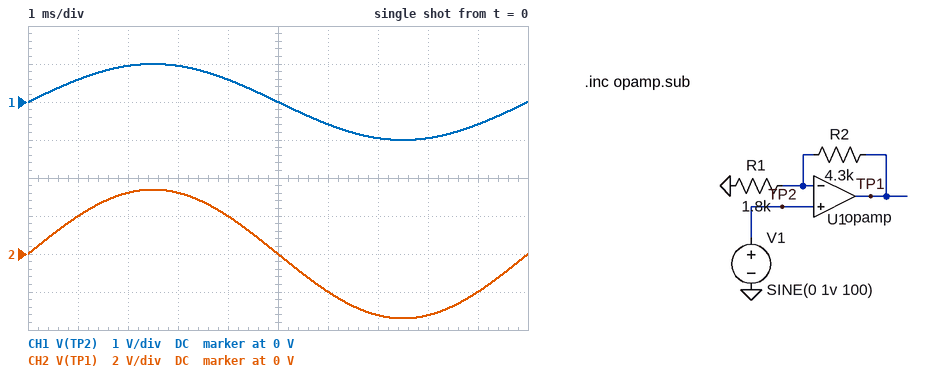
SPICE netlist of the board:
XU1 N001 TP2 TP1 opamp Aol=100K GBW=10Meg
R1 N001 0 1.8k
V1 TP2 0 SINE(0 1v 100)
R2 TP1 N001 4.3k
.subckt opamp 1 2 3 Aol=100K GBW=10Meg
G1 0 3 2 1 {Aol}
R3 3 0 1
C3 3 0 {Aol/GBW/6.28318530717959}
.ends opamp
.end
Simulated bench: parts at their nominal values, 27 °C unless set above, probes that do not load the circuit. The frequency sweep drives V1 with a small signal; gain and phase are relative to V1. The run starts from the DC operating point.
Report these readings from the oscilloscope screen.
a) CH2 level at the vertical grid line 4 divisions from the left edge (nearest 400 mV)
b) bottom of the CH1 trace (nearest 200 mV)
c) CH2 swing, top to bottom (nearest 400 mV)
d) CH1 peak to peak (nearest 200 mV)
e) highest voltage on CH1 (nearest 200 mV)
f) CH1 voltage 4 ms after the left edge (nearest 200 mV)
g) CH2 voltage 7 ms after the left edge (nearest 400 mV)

2.0 V
-1.0 V
6.8 V
2.0 V
1.0 V
600 mV
-3.2 V
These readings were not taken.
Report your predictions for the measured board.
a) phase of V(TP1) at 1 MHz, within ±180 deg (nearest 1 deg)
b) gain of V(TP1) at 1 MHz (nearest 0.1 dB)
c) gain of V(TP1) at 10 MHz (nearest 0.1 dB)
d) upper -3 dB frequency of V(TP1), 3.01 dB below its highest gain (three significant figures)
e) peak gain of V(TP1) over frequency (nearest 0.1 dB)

-19 deg
10.1 dB
-0.4 dB
2.95 MHz
10.6 dB
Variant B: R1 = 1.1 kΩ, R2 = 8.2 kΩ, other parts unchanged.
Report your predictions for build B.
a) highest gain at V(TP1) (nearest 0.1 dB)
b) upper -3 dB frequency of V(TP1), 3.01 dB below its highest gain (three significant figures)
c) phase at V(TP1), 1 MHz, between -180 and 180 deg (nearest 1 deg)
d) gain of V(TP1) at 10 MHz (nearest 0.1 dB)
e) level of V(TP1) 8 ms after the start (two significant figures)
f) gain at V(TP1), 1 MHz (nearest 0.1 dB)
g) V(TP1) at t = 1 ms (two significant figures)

18.5 dB
1.18 MHz
-40 deg
-0.1 dB
-8.0 V
16.2 dB
5.0 V
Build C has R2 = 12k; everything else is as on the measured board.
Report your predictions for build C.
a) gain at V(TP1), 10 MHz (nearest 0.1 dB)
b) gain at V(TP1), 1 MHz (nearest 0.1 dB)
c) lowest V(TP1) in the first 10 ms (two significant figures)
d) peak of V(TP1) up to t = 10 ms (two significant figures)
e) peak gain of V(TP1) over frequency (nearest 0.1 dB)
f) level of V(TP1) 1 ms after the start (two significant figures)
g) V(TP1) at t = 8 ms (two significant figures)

-0.1 dB
15.7 dB
-7.7 V
7.7 V
17.7 dB
4.5 V
-7.3 V
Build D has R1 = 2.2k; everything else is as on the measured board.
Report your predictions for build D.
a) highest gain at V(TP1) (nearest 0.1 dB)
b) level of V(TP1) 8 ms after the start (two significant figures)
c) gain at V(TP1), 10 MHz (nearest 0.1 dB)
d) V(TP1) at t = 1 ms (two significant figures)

9.4 dB
-2.8 V
-0.5 dB
1.7 V
